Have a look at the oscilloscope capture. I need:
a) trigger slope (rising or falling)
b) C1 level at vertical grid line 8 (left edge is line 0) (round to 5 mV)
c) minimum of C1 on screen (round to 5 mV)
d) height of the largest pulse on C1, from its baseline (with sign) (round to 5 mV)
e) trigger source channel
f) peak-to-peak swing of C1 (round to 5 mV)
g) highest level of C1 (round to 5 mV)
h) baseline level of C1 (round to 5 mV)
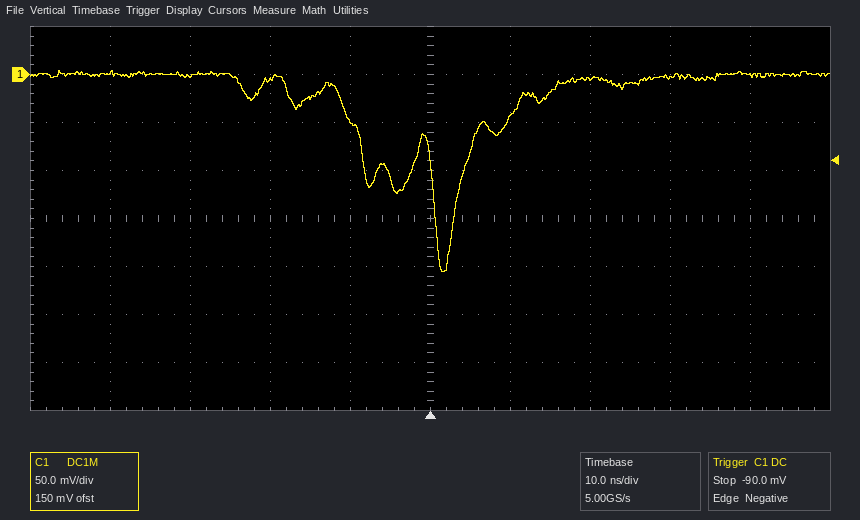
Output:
falling
-5 mV
-205 mV
-205 mV
C1
210 mV
5 mV
0 mV
